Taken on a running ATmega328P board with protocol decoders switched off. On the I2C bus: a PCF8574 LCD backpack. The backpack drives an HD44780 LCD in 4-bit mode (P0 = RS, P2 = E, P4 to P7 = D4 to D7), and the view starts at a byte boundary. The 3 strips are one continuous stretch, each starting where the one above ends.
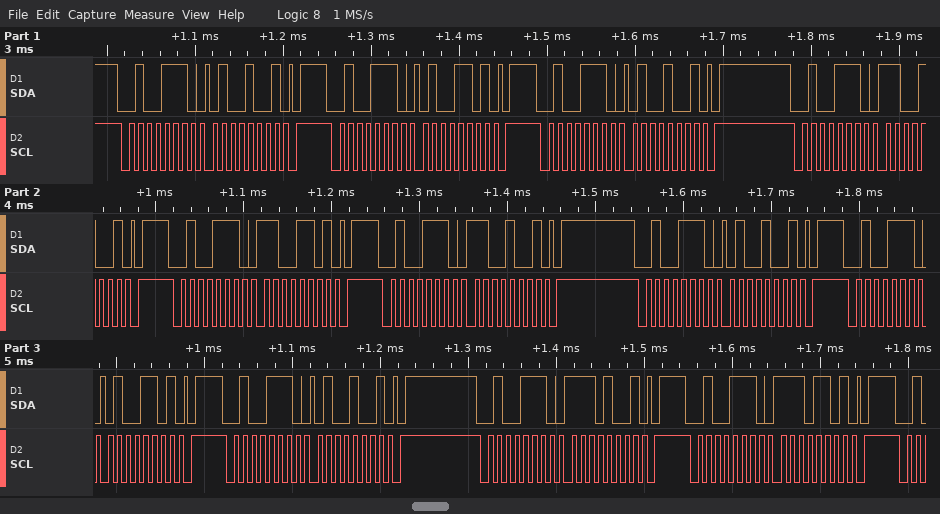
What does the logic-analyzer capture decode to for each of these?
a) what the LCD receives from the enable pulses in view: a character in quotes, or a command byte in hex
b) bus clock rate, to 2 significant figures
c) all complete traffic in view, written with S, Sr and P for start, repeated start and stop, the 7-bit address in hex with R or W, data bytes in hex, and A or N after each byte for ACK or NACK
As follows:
'L'
100 kHz
S 27W A 49 A P S 27W A 4D A P S 27W A 49 A P S 27W A C9 A P S 27W A CD A P S 27W A C9 A P S 27W A 49 A P S 27W A 4D A P S 27W A 49 A P S 27W A E9 A P S 27W A ED A P
